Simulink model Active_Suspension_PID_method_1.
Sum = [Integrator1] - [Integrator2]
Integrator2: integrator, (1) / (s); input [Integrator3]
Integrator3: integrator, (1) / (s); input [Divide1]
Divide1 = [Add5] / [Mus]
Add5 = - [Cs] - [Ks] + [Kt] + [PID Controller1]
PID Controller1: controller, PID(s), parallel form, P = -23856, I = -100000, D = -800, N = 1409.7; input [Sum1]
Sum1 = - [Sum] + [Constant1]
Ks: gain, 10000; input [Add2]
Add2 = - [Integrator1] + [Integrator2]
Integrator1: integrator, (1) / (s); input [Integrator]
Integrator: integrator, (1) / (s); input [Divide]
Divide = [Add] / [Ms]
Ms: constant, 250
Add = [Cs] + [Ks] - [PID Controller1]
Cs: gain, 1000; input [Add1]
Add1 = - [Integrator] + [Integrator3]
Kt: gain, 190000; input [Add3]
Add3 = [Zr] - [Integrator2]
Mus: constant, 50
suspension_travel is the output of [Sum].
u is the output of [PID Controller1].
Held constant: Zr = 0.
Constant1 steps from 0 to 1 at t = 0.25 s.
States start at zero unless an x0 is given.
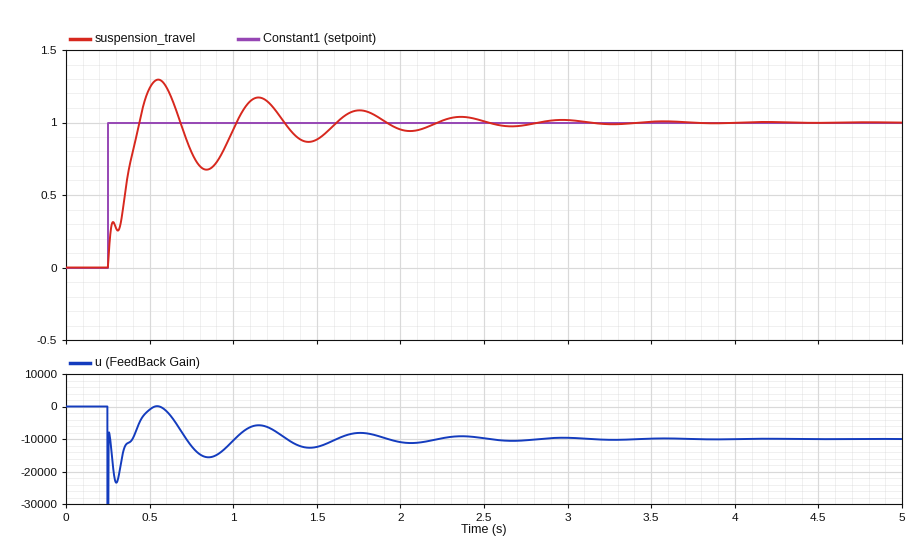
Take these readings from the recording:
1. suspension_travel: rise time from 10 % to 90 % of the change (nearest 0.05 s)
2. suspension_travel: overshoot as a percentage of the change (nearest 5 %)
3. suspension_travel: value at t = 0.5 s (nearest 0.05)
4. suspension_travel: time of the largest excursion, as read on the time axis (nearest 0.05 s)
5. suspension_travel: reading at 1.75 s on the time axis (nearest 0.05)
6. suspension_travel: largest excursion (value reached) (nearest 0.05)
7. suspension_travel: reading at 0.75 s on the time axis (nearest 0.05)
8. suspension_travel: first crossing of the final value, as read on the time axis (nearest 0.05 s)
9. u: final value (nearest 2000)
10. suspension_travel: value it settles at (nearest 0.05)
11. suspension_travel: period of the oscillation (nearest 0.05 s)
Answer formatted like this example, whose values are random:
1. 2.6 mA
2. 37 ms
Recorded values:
1. 0.15 s
2. 30 %
3. 1.25
4. 0.55 s
5. 1.10
6. 1.30
7. 0.80
8. 0.45 s
9. -10000
10. 1.00
11. 0.60 s
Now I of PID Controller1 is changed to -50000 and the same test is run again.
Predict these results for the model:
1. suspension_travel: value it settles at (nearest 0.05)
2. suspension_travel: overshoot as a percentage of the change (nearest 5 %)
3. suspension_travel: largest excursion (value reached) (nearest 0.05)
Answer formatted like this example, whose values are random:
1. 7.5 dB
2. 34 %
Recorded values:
1. 1.00
2. 15 %
3. 1.15
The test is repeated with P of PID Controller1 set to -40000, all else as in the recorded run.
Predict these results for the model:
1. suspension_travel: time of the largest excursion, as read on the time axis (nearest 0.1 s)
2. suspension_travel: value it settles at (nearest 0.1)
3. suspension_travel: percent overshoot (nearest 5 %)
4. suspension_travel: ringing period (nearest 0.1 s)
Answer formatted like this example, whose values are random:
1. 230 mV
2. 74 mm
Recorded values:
1. 0.5 s
2. 1.0
3. 35 %
4. 0.5 s
